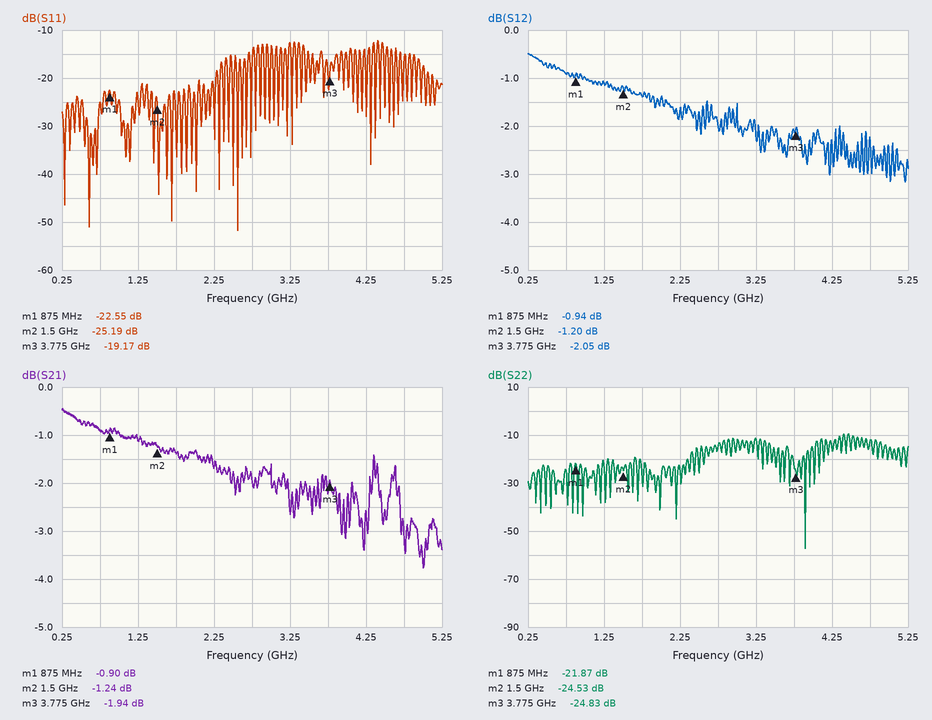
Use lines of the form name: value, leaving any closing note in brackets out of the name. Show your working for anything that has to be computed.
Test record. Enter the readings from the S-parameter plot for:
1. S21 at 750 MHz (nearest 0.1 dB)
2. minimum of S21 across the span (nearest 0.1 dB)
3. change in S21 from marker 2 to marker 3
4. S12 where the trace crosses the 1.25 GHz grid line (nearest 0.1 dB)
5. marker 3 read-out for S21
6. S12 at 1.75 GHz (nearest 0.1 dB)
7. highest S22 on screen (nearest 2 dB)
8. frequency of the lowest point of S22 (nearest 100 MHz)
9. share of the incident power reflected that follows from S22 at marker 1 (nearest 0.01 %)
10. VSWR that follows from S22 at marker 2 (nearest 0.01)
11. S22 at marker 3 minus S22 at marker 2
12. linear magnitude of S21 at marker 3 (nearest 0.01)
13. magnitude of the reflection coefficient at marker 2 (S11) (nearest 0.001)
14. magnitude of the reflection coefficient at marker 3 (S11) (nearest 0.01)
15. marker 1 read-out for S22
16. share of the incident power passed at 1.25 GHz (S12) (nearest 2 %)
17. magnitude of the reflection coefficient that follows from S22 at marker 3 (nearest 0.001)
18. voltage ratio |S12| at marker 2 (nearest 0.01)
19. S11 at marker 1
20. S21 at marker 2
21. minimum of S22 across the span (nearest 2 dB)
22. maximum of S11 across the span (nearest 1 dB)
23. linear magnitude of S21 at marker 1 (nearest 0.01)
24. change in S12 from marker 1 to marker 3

S21 at 750 MHz: -0.9 dB
minimum of S21 across the span: -3.8 dB
change in S21 from marker 2 to marker 3: -1.94 − (-1.24) = -0.70 dB
S12 where the trace crosses the 1.25 GHz grid line: -1.1 dB
marker 3 read-out for S21: -1.94 dB
S12 at 1.75 GHz: -1.4 dB
highest S22 on screen: -10 dB
frequency of the lowest point of S22: 3.9 GHz
share of the incident power reflected that follows from S22 at marker 1: 10^(-21.87/10) ≈ 0.65 %
VSWR that follows from S22 at marker 2: (1 + 0.0594)/(1 − 0.0594) ≈ 1.13
S22 at marker 3 minus S22 at marker 2: -24.83 − (-24.53) = -0.30 dB
linear magnitude of S21 at marker 3: 10^(-1.94/20) ≈ 0.80
magnitude of the reflection coefficient at marker 2 (S11): 10^(-25.19/20) ≈ 0.055
magnitude of the reflection coefficient at marker 3 (S11): 10^(-19.17/20) ≈ 0.11
marker 1 read-out for S22: -21.87 dB
share of the incident power passed at 1.25 GHz (S12): 10^(-1.1/10) ≈ 78 %
magnitude of the reflection coefficient that follows from S22 at marker 3: 10^(-24.83/20) ≈ 0.057
voltage ratio |S12| at marker 2: 10^(-1.2/20) ≈ 0.87
S11 at marker 1: -22.55 dB
S21 at marker 2: -1.24 dB
minimum of S22 across the span: -58 dB
maximum of S11 across the span: -12 dB
linear magnitude of S21 at marker 1: 10^(-0.9/20) ≈ 0.90
change in S12 from marker 1 to marker 3: -2.05 − (-0.94) = -1.11 dB
